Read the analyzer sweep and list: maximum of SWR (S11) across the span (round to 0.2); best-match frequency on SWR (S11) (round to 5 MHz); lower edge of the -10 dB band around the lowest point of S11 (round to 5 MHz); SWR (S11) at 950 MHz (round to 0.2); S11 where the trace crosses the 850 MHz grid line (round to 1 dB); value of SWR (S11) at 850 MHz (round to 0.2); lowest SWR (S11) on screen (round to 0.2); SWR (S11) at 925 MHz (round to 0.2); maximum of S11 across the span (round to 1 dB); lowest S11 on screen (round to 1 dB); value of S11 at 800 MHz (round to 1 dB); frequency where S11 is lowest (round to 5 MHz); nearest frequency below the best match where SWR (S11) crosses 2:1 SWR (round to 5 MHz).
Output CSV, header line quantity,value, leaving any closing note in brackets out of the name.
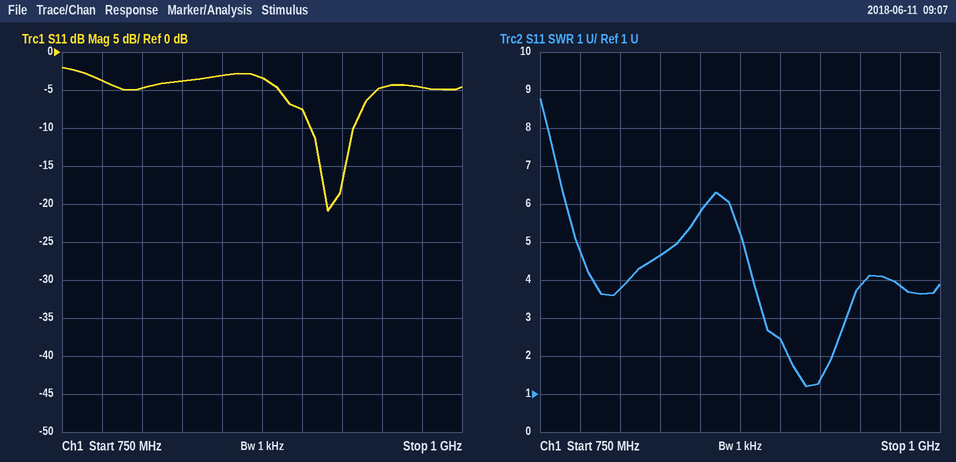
quantity,value
maximum of SWR (S11) across the span,8.8
best-match frequency on SWR (S11),915 MHz
lower edge of the -10 dB band around the lowest point of S11,905 MHz
SWR (S11) at 950 MHz,3.8
S11 where the trace crosses the 850 MHz grid line,-3 dB
value of SWR (S11) at 850 MHz,5.8
lowest SWR (S11) on screen,1.2
SWR (S11) at 925 MHz,1.4
maximum of S11 across the span,-2 dB
lowest S11 on screen,-21 dB
value of S11 at 800 MHz,-5 dB
frequency where S11 is lowest,915 MHz
nearest frequency below the best match where SWR (S11) crosses 2:1 SWR,905 MHz
